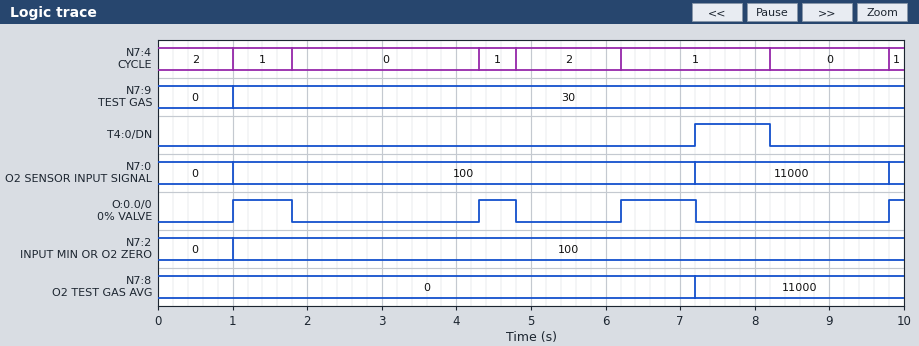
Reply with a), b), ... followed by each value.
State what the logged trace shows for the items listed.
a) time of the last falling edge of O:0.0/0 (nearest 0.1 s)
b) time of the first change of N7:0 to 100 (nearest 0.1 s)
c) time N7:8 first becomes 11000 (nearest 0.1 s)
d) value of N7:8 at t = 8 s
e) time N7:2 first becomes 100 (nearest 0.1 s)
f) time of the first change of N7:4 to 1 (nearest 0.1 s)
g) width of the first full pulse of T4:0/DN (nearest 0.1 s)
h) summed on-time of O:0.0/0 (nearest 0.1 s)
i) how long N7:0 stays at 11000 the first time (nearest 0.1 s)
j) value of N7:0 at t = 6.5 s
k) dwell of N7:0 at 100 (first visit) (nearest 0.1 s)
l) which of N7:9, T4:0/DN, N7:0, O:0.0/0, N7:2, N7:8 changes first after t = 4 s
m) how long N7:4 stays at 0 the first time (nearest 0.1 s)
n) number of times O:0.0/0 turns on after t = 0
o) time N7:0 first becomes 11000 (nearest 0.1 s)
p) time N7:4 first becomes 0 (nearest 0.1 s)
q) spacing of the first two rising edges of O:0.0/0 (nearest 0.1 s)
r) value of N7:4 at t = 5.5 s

a) 7.2 s
b) 1.0 s
c) 7.2 s
d) 11000
e) 1.0 s
f) 1.0 s
g) 1.0 s
h) 2.5 s
i) 2.6 s
j) 100
k) 6.2 s
l) O:0.0/0
m) 2.5 s
n) 4
o) 7.2 s
p) 1.8 s
q) 3.3 s
r) 2
